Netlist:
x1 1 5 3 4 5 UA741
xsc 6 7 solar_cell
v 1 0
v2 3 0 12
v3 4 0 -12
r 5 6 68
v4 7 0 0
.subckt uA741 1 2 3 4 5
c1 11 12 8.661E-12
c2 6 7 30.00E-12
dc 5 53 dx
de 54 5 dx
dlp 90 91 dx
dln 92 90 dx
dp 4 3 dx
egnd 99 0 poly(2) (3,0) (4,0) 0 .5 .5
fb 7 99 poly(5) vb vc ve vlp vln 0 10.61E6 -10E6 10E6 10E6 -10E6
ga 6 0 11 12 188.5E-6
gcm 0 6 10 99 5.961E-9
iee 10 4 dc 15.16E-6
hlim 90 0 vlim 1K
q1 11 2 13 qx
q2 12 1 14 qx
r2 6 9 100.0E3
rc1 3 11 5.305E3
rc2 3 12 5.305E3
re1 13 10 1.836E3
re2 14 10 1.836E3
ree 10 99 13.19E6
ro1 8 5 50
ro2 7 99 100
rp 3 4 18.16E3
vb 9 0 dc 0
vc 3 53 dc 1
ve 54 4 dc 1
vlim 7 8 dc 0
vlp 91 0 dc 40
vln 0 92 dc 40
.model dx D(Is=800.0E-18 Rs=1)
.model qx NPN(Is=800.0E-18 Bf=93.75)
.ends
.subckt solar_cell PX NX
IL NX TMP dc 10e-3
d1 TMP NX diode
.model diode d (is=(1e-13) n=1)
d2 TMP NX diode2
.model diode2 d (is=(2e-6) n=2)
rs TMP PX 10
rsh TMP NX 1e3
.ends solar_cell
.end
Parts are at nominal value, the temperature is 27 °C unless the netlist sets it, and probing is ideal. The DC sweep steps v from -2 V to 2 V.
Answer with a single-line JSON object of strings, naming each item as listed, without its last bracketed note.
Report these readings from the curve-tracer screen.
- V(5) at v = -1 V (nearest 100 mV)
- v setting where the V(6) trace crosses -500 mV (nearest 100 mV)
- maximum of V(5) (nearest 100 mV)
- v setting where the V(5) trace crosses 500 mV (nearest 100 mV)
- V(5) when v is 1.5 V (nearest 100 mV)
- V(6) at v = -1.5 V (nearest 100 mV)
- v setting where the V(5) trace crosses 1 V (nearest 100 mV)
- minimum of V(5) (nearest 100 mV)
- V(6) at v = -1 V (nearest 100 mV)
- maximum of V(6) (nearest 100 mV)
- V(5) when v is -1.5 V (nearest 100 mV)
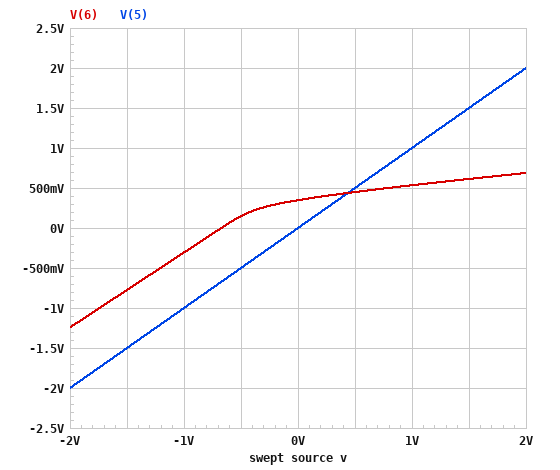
{"V(5) at v = -1 V": "-1.0 V", "v setting where the V(6) trace crosses -500 mV": "-1.2 V", "maximum of V(5)": "2.0 V", "v setting where the V(5) trace crosses 500 mV": "500 mV", "V(5) when v is 1.5 V": "1.5 V", "V(6) at v = -1.5 V": "-800 mV", "v setting where the V(5) trace crosses 1 V": "1.0 V", "minimum of V(5)": "-2.0 V", "V(6) at v = -1 V": "-300 mV", "maximum of V(6)": "700 mV", "V(5) when v is -1.5 V": "-1.5 V"}
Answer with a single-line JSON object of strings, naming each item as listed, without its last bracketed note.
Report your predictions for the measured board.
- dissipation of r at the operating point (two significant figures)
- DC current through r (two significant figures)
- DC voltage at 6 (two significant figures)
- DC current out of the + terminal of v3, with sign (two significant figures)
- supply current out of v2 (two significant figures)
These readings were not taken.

{"dissipation of r at the operating point": "1.8 mW", "DC current through r": "5.1 mA", "DC voltage at 6": "350 mV", "DC current out of the + terminal of v3, with sign": "-1.3 mA", "supply current out of v2": "1.3 mA"}
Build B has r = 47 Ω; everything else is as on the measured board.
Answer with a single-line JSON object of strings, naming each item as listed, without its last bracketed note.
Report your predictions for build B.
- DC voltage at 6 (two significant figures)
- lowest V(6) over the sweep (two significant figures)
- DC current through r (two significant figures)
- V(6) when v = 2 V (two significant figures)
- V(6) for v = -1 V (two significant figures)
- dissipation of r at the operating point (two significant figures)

{"DC voltage at 6": "310 mV", "lowest V(6) over the sweep": "-1.5 V", "DC current through r": "6.6 mA", "V(6) when v = 2 V": "770 mV", "V(6) for v = -1 V": "-510 mV", "dissipation of r at the operating point": "2.1 mW"}
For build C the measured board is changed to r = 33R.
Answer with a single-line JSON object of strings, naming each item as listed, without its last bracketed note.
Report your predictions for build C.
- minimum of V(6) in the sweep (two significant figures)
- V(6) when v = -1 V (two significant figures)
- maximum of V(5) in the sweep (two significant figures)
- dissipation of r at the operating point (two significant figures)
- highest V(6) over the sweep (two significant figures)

{"minimum of V(6) in the sweep": "-1.6 V", "V(6) when v = -1 V": "-650 mV", "maximum of V(5) in the sweep": "2.0 V", "dissipation of r at the operating point": "2.1 mW", "highest V(6) over the sweep": "860 mV"}
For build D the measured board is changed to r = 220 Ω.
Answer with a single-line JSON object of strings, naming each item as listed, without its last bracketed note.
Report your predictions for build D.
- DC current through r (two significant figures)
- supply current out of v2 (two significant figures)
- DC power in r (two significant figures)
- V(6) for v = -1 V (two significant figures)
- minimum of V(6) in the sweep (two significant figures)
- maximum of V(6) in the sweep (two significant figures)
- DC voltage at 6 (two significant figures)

{"DC current through r": "1.9 mA", "supply current out of v2": "1.3 mA", "DC power in r": "760 µW", "V(6) for v = -1 V": "330 mV", "minimum of V(6) in the sweep": "120 mV", "maximum of V(6) in the sweep": "530 mV", "DC voltage at 6": "410 mV"}
